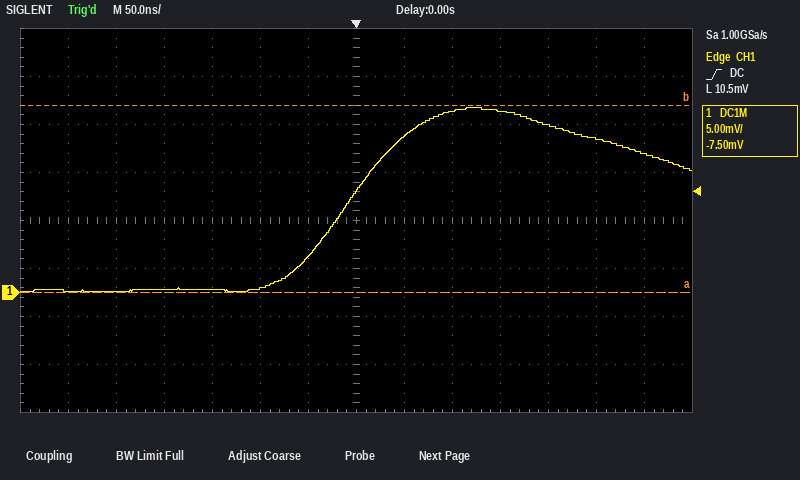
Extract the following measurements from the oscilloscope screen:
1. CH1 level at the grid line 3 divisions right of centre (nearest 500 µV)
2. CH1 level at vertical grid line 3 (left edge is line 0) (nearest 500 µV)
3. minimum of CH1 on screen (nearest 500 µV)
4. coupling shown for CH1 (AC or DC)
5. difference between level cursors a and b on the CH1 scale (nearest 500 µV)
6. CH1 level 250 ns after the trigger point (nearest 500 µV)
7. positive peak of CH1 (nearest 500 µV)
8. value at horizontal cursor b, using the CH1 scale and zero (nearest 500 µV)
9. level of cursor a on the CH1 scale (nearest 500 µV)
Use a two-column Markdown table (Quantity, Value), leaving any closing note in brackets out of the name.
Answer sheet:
| Quantity | Value |
|---|---|
| CH1 level at the grid line 3 divisions right of centre | 19.0 mV |
| CH1 level at vertical grid line 3 (left edge is line 0) | 500 µV |
| minimum of CH1 on screen | 0.0 mV |
| coupling shown for CH1 | DC |
| difference between level cursors a and b on the CH1 scale | 19.5 mV |
| CH1 level 250 ns after the trigger point | 16.0 mV |
| positive peak of CH1 | 19.5 mV |
| value at horizontal cursor b, using the CH1 scale and zero | 19.5 mV |
| level of cursor a on the CH1 scale | 0.0 mV |
